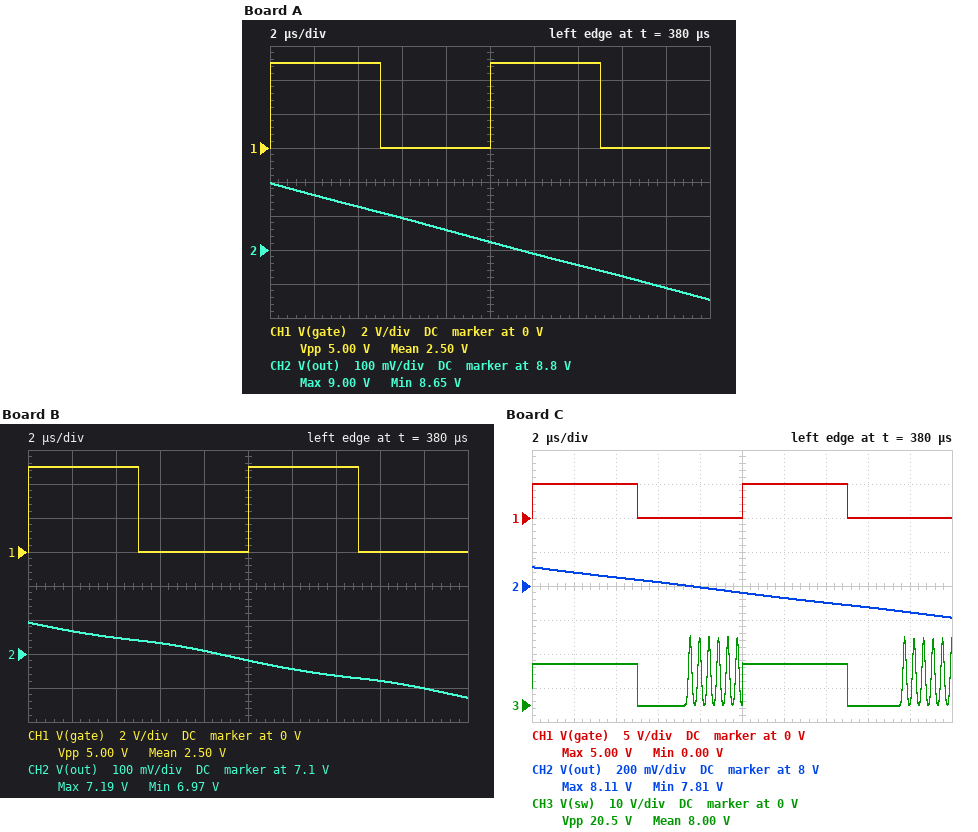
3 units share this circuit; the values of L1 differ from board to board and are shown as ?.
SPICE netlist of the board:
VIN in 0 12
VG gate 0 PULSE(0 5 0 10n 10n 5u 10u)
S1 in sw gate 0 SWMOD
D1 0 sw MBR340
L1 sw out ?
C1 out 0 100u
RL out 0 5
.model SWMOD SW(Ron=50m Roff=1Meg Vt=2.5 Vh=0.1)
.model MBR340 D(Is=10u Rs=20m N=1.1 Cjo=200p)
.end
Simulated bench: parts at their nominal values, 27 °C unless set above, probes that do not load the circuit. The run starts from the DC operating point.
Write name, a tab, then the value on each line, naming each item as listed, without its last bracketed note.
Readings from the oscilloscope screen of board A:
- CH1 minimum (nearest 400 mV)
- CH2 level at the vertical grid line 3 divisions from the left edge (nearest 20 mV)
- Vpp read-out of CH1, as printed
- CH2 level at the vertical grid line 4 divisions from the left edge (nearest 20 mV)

CH1 minimum	0 V
CH2 level at the vertical grid line 3 divisions from the left edge	8.90 V
Vpp read-out of CH1, as printed	5.00 V
CH2 level at the vertical grid line 4 divisions from the left edge	8.86 V
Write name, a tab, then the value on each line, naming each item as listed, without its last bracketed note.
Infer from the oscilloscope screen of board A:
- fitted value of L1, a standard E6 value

fitted value of L1, a standard E6 value	100 µH
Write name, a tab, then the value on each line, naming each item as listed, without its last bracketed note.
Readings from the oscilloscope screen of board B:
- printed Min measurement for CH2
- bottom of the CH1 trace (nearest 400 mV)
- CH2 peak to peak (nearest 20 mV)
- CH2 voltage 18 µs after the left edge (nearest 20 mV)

printed Min measurement for CH2	6.97 V
bottom of the CH1 trace	0 V
CH2 peak to peak	220 mV
CH2 voltage 18 µs after the left edge	7.00 V
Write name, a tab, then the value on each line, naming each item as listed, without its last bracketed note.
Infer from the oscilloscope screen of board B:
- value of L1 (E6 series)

value of L1	33 µH
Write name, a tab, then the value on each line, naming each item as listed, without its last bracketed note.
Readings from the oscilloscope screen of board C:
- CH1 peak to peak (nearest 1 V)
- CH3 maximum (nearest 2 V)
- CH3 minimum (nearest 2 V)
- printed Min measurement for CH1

CH1 peak to peak	5 V
CH3 maximum	20 V
CH3 minimum	0 V
printed Min measurement for CH1	0.00 V
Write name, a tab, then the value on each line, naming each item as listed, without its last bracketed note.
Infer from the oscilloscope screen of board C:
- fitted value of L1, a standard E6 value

fitted value of L1, a standard E6 value	68 µH
